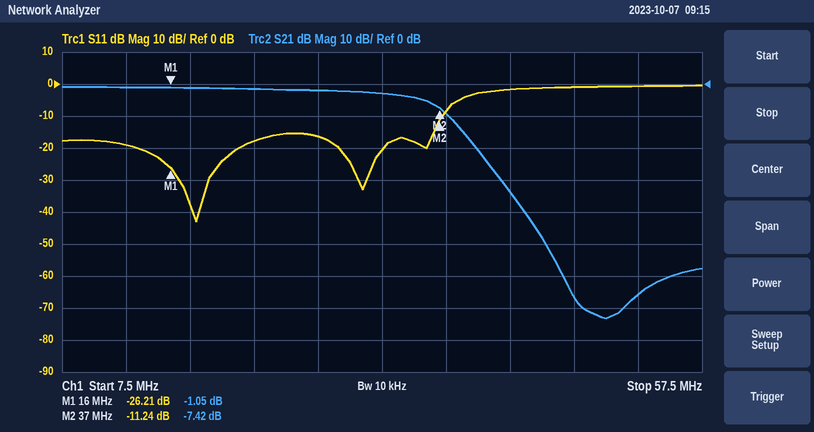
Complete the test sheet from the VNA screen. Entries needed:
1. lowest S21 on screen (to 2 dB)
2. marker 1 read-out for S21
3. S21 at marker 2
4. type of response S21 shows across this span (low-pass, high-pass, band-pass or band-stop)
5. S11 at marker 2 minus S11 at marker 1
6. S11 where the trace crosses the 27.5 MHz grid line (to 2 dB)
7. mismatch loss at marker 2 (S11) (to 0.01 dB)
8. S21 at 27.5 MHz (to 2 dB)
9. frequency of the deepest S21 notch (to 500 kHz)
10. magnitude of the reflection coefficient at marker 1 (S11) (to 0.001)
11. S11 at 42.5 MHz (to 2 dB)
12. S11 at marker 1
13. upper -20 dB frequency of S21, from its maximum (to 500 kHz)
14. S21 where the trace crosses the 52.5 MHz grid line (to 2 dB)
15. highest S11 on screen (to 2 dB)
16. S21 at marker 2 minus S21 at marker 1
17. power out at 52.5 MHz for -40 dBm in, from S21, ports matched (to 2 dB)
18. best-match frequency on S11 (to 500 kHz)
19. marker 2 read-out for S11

-74 dB
-1.05 dB
-7.42 dB
low-pass
14.97 dB
-16 dB
0.34 dB
-2 dB
50.0 MHz
0.049
-2 dB
-26.21 dB
40.0 MHz
-66 dB
0 dB
-6.37 dB
-106 dBm
18.0 MHz
-11.24 dB
